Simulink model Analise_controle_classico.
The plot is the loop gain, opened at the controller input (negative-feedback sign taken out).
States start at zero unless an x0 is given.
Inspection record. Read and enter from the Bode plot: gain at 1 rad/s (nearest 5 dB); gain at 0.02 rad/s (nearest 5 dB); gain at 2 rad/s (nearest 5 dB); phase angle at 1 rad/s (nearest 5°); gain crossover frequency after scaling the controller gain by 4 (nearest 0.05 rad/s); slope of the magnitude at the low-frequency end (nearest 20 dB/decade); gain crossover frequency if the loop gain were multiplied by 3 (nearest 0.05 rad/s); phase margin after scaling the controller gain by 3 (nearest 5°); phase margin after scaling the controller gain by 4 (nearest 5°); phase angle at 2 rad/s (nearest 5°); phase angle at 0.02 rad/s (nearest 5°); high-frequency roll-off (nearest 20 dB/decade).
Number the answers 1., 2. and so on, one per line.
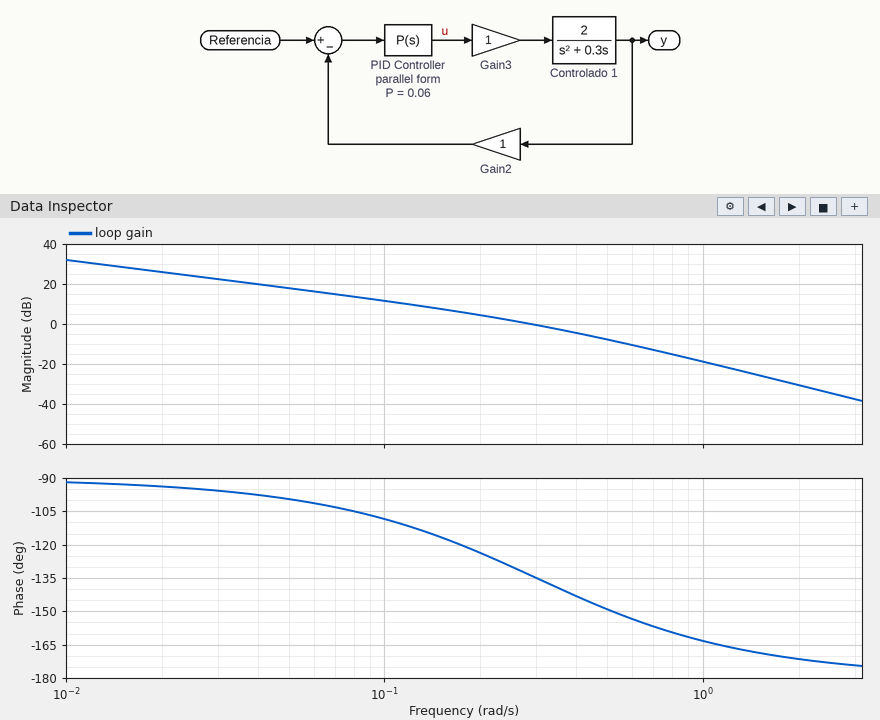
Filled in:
1. -20 dB
2. 25 dB
3. -30 dB
4. -165°
5. 0.65 rad/s
6. -20 dB/decade
7. 0.55 rad/s
8. 30°
9. 25°
10. -170°
11. -95°
12. -40 dB/decade
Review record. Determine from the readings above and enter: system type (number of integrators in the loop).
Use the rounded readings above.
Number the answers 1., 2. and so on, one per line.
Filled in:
1. 1
